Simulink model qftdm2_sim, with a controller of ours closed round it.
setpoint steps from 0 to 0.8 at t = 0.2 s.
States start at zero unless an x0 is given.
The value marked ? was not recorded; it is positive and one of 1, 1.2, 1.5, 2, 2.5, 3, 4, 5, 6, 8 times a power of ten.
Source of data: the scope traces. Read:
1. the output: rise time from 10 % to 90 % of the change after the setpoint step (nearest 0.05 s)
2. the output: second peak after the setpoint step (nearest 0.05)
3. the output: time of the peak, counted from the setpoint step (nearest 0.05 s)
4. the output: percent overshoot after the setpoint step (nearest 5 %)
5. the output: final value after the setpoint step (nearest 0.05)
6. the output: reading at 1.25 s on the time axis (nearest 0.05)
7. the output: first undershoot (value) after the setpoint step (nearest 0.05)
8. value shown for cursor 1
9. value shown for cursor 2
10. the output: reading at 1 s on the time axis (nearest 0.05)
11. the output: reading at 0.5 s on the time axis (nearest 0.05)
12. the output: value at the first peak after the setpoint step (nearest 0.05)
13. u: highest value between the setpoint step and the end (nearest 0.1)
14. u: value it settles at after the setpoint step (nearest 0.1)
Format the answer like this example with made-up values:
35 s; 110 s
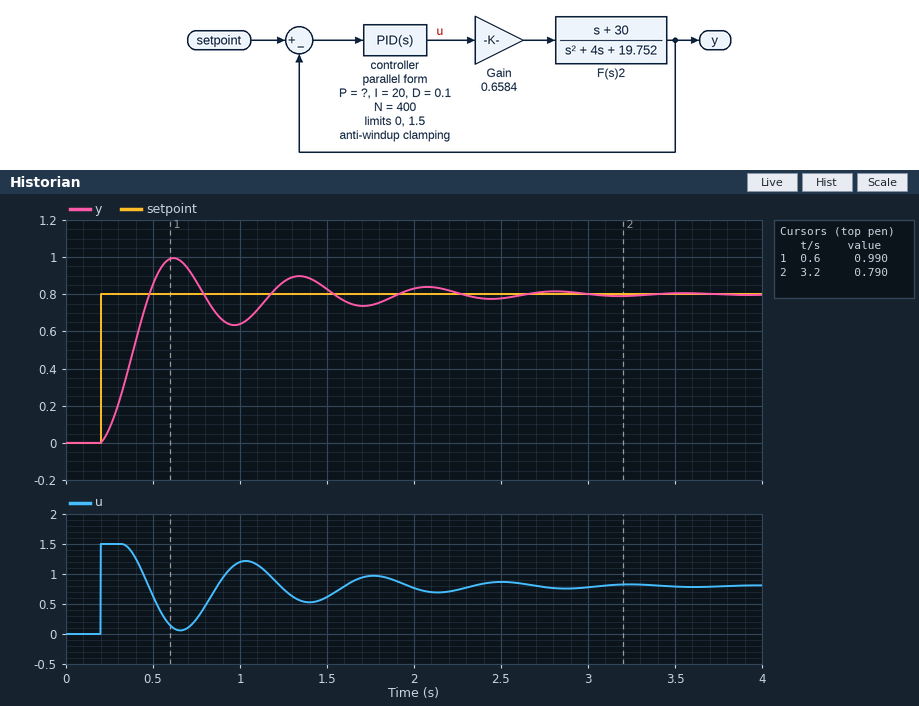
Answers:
0.20 s; 0.90; 0.40 s; 25 %; 0.80; 0.85; 0.65; 0.990; 0.790; 0.65; 0.85; 1.00; 1.5; 0.8
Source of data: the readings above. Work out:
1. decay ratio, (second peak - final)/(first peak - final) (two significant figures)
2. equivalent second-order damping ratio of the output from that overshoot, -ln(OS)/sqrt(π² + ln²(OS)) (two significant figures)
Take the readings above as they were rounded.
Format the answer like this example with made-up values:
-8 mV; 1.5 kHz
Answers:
0.50; 0.40
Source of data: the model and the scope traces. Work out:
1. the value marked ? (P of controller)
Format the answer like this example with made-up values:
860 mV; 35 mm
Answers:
3
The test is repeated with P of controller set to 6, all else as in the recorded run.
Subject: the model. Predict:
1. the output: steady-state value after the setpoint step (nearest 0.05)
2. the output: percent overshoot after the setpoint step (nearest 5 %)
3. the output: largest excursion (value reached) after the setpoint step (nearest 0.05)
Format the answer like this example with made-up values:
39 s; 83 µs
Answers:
0.80; 10 %; 0.85
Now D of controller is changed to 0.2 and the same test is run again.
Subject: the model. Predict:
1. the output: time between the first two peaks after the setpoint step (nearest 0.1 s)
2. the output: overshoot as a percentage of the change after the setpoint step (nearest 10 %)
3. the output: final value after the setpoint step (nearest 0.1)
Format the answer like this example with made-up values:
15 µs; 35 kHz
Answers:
0.8 s; 30 %; 0.8
